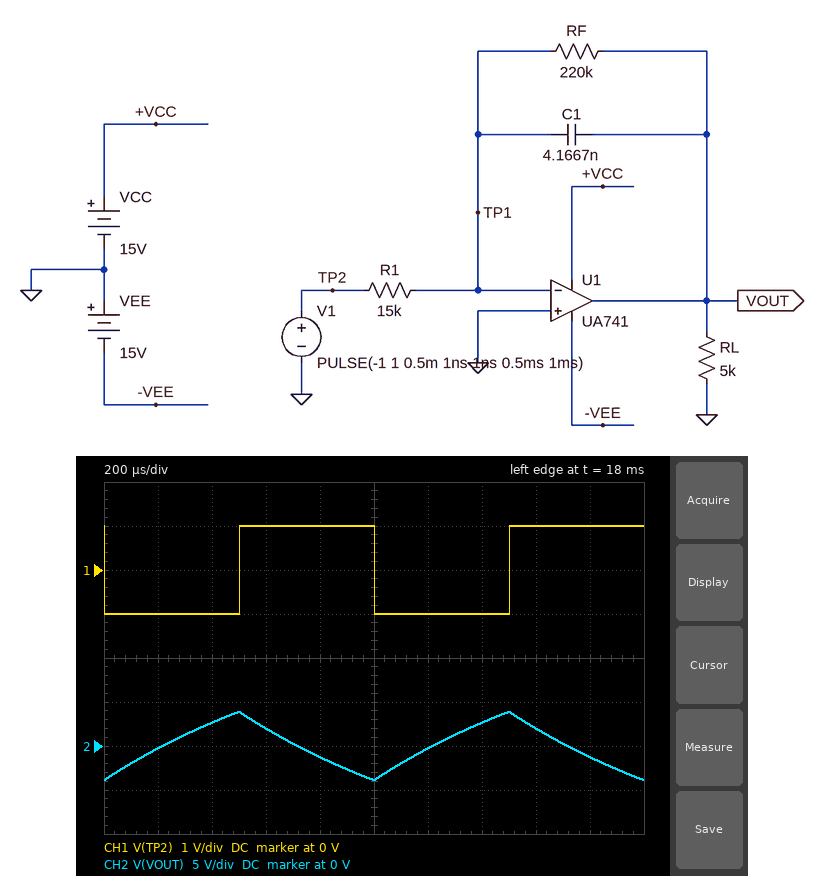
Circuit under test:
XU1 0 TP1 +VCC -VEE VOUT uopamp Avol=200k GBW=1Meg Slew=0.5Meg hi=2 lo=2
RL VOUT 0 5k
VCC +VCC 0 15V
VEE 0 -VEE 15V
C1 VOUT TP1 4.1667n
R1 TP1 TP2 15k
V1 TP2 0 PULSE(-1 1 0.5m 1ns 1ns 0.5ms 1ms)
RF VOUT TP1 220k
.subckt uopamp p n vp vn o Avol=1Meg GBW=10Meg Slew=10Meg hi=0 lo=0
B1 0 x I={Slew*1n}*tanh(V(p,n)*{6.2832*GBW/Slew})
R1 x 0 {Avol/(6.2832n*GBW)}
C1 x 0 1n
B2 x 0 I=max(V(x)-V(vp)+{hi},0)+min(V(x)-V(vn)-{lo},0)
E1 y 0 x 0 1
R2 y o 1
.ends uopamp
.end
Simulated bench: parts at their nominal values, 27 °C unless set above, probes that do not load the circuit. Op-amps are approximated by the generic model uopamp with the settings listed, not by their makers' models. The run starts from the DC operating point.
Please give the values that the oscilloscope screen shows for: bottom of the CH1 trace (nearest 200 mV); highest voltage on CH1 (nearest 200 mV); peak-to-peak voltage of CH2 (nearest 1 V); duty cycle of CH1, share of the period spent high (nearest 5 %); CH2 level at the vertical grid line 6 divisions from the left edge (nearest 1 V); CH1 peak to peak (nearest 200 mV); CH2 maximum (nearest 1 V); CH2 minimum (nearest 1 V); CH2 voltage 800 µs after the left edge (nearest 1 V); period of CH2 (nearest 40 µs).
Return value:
-1.0 V
1.0 V
8 V
50 %
0 V
2.0 V
4 V
-4 V
-1 V
1.00 ms
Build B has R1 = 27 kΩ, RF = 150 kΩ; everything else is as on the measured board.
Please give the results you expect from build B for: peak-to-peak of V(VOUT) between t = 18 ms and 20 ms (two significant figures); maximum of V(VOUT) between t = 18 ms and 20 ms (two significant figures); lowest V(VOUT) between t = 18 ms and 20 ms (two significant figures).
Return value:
4.2 V
2.1 V
-2.1 V
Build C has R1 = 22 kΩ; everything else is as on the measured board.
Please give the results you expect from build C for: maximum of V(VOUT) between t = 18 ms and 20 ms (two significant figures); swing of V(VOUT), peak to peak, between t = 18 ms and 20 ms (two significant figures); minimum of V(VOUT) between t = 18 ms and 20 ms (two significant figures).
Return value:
2.7 V
5.3 V
-2.7 V
